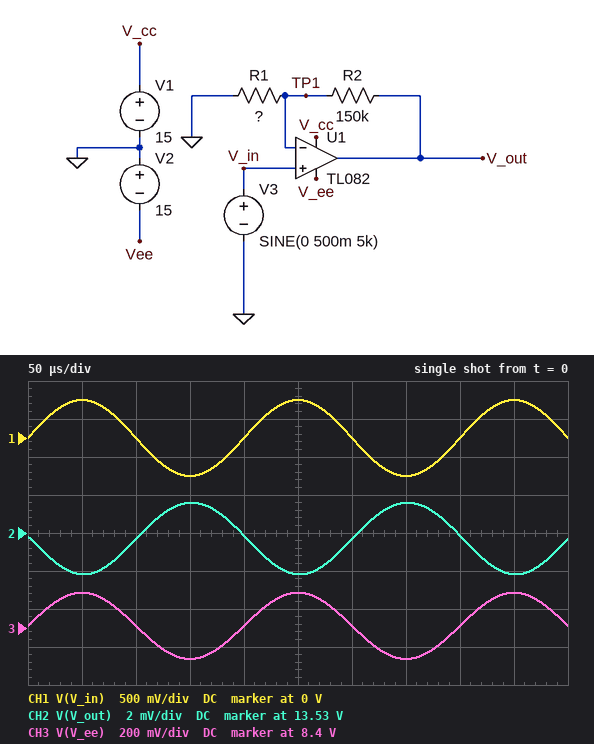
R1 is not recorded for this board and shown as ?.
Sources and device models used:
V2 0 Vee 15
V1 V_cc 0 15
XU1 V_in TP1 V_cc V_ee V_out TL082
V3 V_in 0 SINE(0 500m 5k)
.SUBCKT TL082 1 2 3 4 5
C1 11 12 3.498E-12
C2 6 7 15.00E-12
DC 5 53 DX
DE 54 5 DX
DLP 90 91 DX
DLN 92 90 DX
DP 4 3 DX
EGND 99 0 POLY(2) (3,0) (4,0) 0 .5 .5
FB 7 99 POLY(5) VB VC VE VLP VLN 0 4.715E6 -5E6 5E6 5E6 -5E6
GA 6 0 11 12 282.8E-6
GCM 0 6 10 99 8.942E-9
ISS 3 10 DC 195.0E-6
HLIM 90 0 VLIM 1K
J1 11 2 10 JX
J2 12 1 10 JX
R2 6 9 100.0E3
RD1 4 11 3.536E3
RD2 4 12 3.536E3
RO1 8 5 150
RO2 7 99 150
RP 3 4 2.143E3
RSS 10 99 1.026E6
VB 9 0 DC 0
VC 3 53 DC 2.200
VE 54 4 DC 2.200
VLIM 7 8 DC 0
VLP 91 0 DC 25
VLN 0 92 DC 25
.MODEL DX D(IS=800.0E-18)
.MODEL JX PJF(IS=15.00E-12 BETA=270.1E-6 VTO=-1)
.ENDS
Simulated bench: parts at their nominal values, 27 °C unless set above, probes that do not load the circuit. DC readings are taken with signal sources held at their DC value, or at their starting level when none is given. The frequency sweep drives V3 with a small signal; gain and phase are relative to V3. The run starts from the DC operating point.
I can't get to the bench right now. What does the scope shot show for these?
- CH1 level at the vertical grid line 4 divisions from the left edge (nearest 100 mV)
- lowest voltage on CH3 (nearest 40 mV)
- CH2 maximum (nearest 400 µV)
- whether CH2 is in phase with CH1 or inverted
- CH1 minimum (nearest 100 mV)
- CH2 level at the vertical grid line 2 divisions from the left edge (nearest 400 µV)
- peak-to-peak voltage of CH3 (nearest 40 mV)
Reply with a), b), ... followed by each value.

a) 0 V
b) 8.24 V
c) 13.5296 V
d) inverted
e) -500 mV
f) 13.5276 V
g) 360 mV
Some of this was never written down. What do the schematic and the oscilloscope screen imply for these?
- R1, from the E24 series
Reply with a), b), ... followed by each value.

a) 15 kΩ
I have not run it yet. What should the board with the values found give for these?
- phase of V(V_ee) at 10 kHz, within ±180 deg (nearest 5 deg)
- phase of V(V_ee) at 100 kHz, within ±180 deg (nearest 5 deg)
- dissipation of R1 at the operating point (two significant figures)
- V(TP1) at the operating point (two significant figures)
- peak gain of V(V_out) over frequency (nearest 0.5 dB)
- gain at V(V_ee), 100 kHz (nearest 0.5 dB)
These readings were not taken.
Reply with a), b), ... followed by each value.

a) 0 deg
b) 0 deg
c) 1.7 mW
d) 5.0 V
e) -48.5 dB
f) -9.0 dB
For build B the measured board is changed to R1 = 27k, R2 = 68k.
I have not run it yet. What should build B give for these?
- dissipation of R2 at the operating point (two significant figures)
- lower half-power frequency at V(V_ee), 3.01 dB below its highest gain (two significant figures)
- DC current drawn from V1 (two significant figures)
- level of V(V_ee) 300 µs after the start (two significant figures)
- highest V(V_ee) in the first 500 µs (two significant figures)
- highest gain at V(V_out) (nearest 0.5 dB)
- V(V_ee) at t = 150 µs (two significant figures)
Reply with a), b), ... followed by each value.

a) 840 µW
b) 4.9 MHz
c) 1.6 mA
d) 8.7 V
e) 8.8 V
f) -50.0 dB
g) 8.5 V
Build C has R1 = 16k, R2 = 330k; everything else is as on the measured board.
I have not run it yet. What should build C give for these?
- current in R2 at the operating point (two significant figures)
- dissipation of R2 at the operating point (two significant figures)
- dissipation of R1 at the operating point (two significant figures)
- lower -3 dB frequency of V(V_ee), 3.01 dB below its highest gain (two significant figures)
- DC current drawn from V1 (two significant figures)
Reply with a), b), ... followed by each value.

a) 26 µA
b) 220 µW
c) 1.6 mW
d) 5.2 MHz
e) 2.0 mA
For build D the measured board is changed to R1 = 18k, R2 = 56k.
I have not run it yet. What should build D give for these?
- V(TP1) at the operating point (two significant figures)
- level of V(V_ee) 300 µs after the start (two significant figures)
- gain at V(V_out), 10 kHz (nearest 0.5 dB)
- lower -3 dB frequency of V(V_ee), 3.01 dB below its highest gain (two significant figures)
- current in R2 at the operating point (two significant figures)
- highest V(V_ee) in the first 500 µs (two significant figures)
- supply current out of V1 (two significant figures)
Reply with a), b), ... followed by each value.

a) 5.6 V
b) 8.6 V
c) -49.5 dB
d) 5.7 MHz
e) 140 µA
f) 8.7 V
g) 1.7 mA
